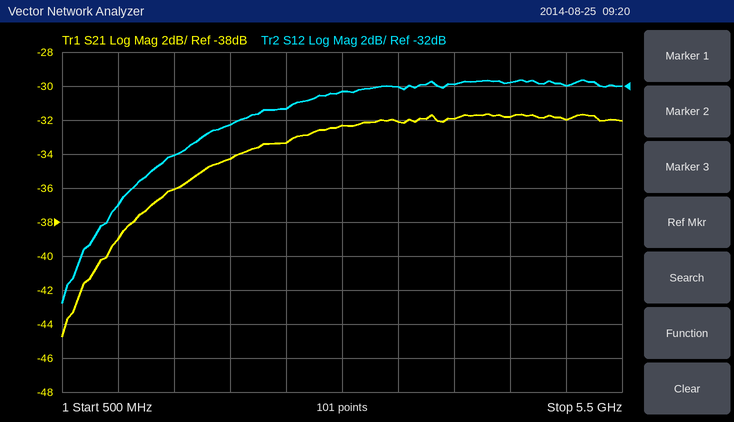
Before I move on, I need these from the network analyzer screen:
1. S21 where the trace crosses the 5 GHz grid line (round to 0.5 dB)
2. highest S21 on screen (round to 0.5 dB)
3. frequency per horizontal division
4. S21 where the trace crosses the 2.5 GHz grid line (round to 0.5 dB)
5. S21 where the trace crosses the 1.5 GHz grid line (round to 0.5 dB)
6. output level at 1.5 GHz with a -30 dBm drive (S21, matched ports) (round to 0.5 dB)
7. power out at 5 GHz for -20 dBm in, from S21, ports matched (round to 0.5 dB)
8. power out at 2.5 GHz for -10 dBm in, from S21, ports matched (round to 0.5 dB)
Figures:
-32.0 dB
-31.5 dB
500 MHz
-33.5 dB
-36.0 dB
-66.0 dBm
-52.0 dBm
-43.5 dBm
